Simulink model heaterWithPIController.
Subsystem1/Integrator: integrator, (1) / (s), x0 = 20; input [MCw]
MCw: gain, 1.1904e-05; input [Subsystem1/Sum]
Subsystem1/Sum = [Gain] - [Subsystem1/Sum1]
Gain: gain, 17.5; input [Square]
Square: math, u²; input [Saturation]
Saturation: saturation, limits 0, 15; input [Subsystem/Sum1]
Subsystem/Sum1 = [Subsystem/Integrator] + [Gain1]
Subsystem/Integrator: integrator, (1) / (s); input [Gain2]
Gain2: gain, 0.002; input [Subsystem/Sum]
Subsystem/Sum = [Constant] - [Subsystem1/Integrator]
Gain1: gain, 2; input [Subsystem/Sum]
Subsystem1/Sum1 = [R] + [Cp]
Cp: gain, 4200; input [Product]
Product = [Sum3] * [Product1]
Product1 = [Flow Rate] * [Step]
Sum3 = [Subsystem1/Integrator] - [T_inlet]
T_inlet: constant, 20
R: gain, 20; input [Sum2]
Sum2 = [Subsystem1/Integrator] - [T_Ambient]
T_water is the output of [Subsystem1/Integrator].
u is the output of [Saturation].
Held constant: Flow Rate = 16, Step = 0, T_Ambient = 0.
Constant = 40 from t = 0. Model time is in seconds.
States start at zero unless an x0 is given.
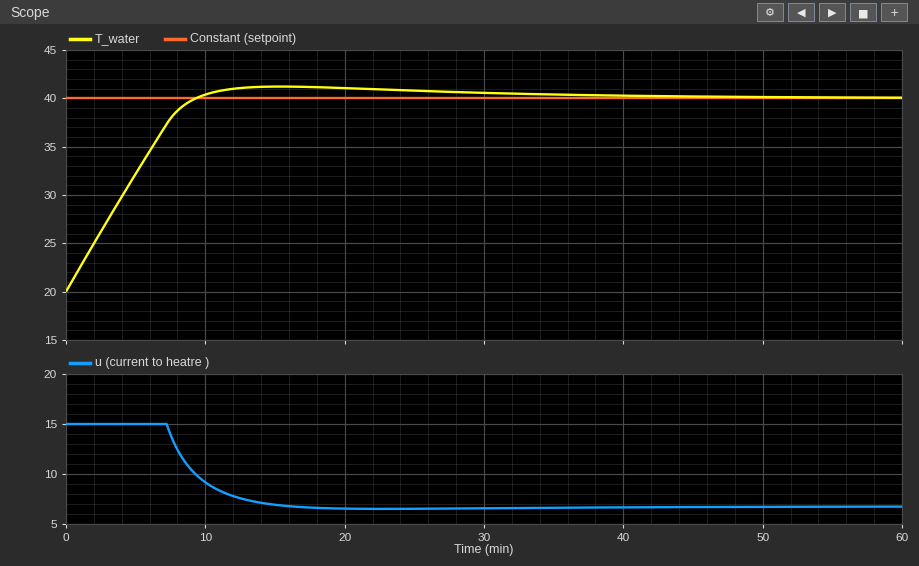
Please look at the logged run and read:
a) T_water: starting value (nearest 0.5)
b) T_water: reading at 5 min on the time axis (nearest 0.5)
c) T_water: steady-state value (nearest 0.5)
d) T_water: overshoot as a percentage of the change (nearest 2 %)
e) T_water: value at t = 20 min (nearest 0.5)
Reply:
20.0
32.0
40.0
6 %
41.0
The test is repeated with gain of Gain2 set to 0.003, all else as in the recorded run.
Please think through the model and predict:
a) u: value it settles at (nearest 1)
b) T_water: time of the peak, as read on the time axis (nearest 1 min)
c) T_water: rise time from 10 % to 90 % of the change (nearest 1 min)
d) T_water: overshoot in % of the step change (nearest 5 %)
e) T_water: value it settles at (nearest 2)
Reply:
7
13 min
7 min
15 %
40
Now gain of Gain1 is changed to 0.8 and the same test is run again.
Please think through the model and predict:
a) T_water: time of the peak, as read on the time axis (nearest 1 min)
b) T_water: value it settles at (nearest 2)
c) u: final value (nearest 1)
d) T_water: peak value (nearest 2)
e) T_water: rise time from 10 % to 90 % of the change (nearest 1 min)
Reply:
18 min
40
7
42
8 min
